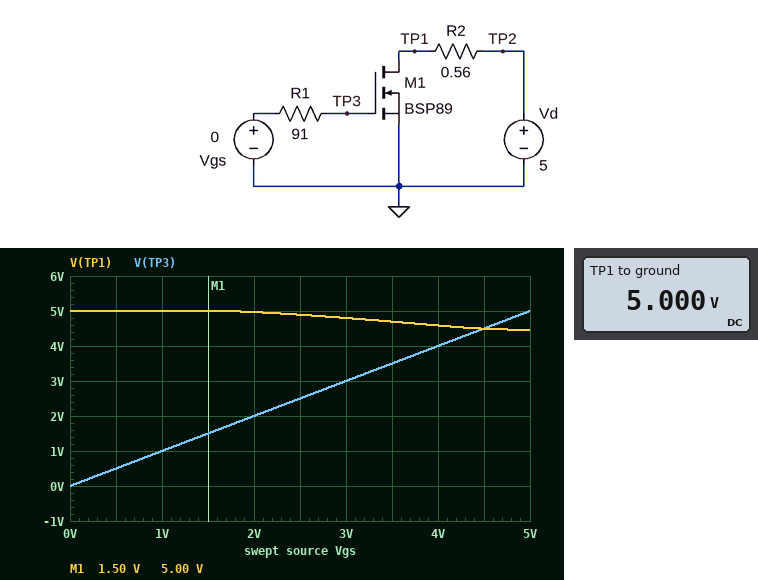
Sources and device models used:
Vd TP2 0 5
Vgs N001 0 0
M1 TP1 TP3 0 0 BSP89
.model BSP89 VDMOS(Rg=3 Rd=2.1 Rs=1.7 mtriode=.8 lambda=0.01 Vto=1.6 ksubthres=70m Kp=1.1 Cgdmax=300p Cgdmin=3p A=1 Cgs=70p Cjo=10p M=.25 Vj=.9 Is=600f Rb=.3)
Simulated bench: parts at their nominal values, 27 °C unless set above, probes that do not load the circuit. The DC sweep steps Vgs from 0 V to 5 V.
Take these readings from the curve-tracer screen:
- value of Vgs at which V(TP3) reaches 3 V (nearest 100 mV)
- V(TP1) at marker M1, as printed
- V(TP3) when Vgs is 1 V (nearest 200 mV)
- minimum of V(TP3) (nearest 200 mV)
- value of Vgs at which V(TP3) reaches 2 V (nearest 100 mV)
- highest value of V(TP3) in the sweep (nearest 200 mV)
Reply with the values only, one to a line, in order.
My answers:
3.0 V
5.00 V
1.0 V
0 V
2.0 V
5.0 V
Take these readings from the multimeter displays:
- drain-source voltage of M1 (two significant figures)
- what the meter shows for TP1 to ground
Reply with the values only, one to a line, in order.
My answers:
5.0 V
5.000 V
